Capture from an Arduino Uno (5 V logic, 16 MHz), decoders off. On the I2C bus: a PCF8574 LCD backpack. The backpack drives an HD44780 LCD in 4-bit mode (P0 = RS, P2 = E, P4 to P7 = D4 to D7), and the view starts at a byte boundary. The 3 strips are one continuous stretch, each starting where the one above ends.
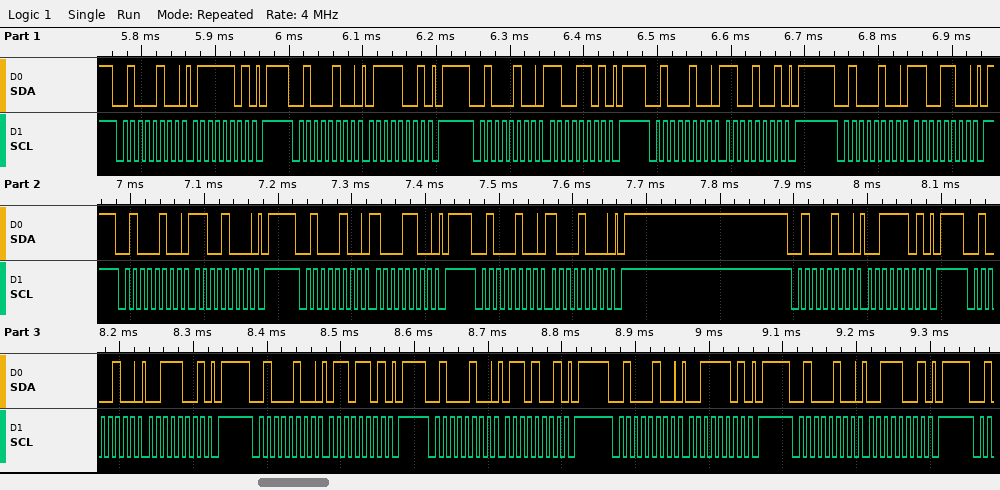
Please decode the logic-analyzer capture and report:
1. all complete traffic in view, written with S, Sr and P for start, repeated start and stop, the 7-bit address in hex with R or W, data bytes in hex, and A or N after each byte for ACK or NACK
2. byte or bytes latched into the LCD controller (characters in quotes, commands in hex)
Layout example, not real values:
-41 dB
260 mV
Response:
S 22W A 7D A P S 22W A 79 A P S 22W A CD A P S 22W A C9 A P S 22W A CC A P S 22W A C8 A P S 22W A 8C A P S 22W A 88 A P S 22W A 3D A P S 22W A 39 A P S 22W A 6D A P S 22W A 69 A P S 22W A 3D A P S 22W A 39 A P
'|' 0xC8 '6'
